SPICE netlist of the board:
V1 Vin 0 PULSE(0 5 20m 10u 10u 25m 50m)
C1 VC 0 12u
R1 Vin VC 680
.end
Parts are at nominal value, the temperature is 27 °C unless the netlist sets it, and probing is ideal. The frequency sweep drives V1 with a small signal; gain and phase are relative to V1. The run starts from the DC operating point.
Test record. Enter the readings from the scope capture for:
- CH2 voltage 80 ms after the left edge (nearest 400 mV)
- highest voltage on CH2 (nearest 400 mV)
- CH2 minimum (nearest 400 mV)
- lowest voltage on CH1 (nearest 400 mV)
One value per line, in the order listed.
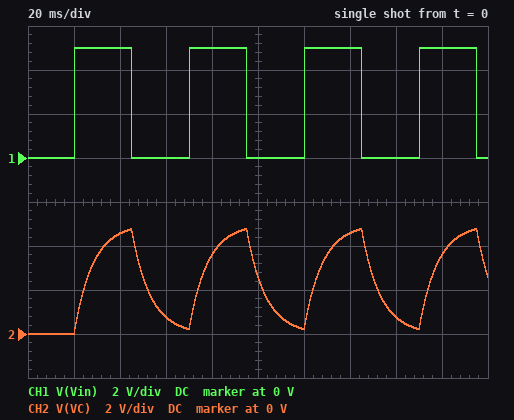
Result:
3.6 V
4.8 V
0 V
0 V
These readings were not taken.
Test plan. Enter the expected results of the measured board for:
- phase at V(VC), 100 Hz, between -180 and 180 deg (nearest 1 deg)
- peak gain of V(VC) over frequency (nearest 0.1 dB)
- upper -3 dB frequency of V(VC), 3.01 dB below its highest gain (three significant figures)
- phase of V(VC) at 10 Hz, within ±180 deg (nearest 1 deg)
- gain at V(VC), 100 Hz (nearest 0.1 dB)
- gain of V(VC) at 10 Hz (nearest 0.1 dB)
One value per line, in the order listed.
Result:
-79 deg
0 dB
19.5 Hz
-27 deg
-14.4 dB
-1.0 dB
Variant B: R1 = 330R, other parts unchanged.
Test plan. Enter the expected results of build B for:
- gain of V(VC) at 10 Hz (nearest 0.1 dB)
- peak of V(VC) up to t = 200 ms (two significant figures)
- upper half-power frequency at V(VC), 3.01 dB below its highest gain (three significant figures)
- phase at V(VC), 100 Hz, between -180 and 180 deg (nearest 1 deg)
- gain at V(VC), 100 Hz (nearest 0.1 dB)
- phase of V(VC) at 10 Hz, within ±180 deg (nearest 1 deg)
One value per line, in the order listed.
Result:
-0.3 dB
5.0 V
40.2 Hz
-68 deg
-8.6 dB
-14 deg
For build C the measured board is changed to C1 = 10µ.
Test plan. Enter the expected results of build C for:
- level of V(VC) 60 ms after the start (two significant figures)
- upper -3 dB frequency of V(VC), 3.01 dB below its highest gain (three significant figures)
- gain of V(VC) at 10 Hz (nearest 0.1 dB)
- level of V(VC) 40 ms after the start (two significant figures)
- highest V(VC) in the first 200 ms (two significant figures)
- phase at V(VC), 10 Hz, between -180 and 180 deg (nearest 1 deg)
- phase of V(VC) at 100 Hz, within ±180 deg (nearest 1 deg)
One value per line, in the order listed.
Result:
540 mV
23.4 Hz
-0.7 dB
4.7 V
4.9 V
-23 deg
-77 deg
